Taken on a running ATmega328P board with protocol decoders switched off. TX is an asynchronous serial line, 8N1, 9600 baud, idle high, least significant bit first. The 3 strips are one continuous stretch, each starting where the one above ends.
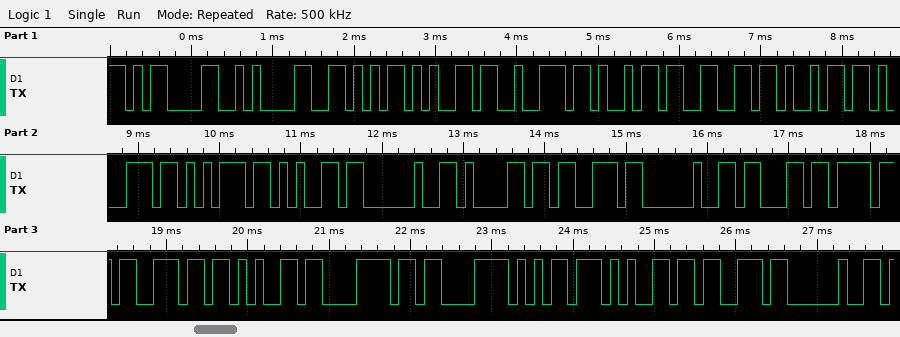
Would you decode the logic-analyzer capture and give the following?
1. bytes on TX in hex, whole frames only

0x0D 0x0A 0x56 0x65 0x72 0x69 0x66 0x69 0x71 0x75 0x65 0x20 0x61 0x73 0x20 0x63 0x6F 0x6E 0x65 0x78 0xC3 0xB5 0x65 0x73 0x20
